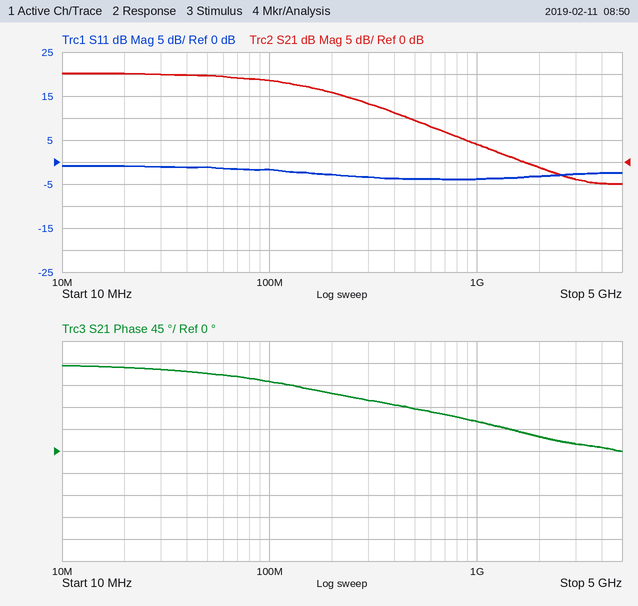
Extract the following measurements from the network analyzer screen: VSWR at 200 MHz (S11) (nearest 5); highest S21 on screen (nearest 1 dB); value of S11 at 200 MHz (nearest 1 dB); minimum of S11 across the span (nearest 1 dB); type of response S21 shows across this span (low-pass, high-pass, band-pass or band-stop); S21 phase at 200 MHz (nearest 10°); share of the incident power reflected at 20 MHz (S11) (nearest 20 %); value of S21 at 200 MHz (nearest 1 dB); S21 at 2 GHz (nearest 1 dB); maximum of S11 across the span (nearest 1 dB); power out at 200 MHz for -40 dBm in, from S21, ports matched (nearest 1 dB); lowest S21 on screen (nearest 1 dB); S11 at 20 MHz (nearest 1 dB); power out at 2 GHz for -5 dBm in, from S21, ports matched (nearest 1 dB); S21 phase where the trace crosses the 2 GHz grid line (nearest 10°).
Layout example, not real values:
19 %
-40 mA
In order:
5
20 dB
-3 dB
-4 dB
low-pass
120°
80 %
16 dB
-1 dB
-1 dB
-24 dBm
-5 dB
-1 dB
-6 dBm
30°
